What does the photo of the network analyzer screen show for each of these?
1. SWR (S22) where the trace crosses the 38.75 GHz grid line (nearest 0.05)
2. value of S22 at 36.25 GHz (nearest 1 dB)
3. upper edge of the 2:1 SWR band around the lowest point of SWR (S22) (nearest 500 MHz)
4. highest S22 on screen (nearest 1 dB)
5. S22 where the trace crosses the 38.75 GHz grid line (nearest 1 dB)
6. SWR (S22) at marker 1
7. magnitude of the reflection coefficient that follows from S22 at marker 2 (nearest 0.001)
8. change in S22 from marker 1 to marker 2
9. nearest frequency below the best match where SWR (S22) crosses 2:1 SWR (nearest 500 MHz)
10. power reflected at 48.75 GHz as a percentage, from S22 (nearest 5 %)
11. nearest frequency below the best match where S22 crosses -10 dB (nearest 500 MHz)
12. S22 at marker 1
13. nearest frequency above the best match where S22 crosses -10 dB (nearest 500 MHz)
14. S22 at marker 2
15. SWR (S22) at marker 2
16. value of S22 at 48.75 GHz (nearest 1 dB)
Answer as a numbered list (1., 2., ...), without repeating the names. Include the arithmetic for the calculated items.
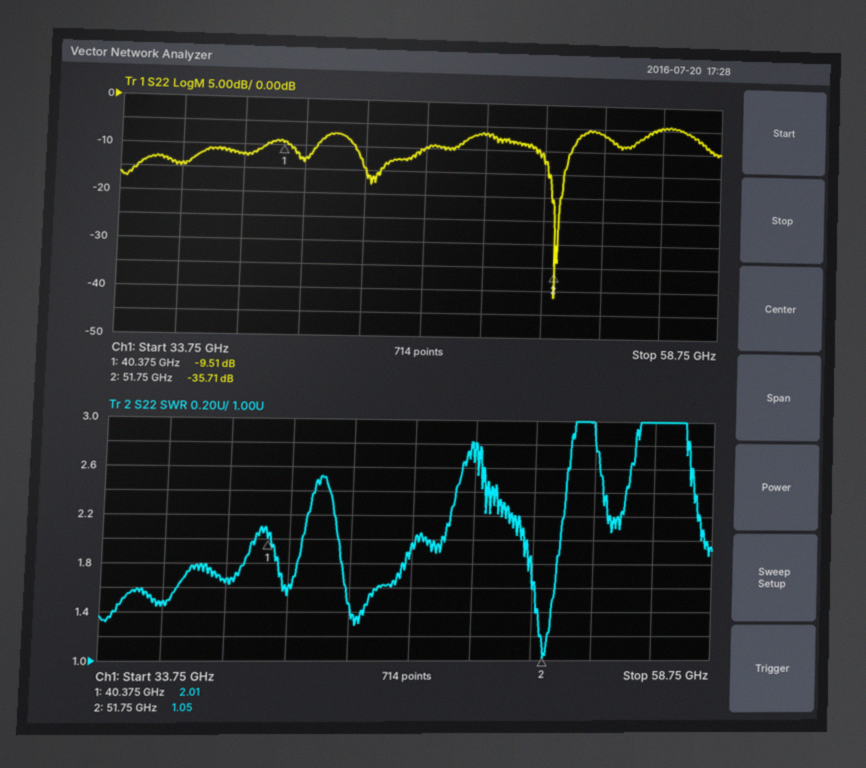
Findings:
1. 1.65
2. -14 dB
3. 52.5 GHz
4. -4 dB
5. -12 dB
6. 2.01
7. 10^(-35.71/20) ≈ 0.016
8. -35.71 − (-9.51) = -26.20 dB
9. 51.0 GHz
10. 10^(-7/10) ≈ 20 %
11. 51.0 GHz
12. -9.51 dB
13. 52.5 GHz
14. -35.71 dB
15. 1.05
16. -7 dB
